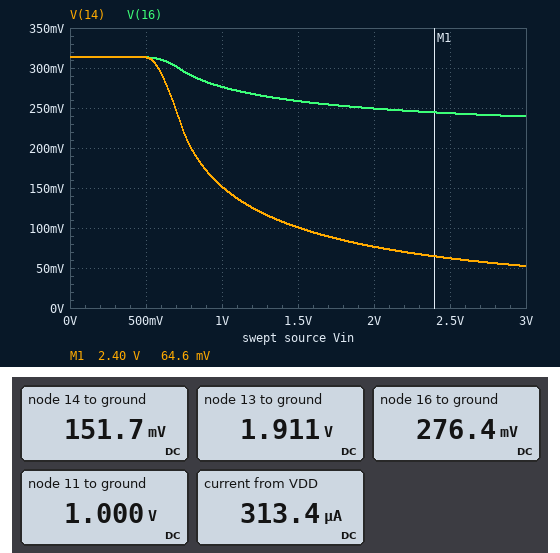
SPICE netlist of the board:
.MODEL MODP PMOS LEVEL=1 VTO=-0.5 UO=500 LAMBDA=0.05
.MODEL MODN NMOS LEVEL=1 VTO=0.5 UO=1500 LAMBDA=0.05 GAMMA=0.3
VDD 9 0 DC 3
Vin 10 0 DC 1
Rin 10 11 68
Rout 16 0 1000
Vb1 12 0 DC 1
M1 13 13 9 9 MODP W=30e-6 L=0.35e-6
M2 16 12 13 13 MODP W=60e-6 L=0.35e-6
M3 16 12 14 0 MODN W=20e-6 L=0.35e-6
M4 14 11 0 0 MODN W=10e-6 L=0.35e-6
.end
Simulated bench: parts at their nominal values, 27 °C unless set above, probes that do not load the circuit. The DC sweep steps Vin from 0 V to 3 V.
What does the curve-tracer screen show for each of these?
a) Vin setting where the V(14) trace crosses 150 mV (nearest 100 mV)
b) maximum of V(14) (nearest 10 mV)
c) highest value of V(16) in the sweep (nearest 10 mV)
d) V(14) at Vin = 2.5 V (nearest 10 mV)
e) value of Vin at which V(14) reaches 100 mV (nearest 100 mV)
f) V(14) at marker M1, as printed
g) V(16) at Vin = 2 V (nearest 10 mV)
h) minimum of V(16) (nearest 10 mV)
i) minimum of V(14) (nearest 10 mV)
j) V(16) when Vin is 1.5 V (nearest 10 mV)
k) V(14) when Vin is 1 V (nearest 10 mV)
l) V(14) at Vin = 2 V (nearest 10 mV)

1.0 V
310 mV
310 mV
60 mV
1.5 V
64.6 mV
250 mV
240 mV
50 mV
260 mV
150 mV
80 mV
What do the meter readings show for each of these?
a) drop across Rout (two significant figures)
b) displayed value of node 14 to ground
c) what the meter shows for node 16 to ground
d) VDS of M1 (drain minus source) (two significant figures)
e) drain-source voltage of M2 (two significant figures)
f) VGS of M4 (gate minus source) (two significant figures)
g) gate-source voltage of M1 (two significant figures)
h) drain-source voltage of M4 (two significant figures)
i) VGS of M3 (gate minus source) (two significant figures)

280 mV
151.7 mV
276.4 mV
-1.1 V
-1.6 V
1.0 V
-1.1 V
150 mV
850 mV
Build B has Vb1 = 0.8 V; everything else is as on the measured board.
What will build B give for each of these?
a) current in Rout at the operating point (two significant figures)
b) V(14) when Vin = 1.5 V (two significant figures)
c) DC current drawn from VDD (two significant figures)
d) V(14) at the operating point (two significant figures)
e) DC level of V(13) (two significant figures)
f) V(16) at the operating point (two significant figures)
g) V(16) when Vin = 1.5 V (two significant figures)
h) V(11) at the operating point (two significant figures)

430 µA
57 mV
450 µA
86 mV
1.8 V
430 mV
420 mV
1.0 V
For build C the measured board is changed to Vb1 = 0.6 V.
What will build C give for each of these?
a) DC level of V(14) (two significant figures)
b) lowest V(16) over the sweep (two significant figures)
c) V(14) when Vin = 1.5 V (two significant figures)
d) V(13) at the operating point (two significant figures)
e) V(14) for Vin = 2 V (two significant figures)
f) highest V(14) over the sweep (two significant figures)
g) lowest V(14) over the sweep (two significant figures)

14 mV
610 mV
8.4 mV
1.7 V
5.9 mV
84 mV
3.8 mV
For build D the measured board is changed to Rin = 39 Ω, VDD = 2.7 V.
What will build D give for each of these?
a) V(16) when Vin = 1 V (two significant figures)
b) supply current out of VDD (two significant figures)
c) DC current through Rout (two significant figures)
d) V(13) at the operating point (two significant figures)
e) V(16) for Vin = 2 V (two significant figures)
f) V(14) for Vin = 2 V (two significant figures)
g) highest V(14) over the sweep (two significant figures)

130 mV
150 µA
130 µA
1.8 V
120 mV
42 mV
150 mV
